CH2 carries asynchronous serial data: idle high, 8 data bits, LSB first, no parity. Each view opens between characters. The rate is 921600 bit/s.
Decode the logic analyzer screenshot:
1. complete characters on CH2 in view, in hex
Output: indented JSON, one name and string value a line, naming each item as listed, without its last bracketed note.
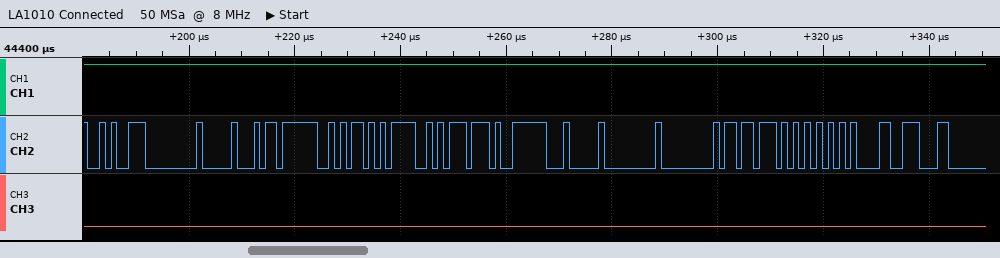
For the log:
{
  "complete characters on CH2 in view, in hex": "CA, 00, 10, FB, 6A, 3D, DD, F9, 04, 00, 00, DB, 55, 85, 8E"
}
